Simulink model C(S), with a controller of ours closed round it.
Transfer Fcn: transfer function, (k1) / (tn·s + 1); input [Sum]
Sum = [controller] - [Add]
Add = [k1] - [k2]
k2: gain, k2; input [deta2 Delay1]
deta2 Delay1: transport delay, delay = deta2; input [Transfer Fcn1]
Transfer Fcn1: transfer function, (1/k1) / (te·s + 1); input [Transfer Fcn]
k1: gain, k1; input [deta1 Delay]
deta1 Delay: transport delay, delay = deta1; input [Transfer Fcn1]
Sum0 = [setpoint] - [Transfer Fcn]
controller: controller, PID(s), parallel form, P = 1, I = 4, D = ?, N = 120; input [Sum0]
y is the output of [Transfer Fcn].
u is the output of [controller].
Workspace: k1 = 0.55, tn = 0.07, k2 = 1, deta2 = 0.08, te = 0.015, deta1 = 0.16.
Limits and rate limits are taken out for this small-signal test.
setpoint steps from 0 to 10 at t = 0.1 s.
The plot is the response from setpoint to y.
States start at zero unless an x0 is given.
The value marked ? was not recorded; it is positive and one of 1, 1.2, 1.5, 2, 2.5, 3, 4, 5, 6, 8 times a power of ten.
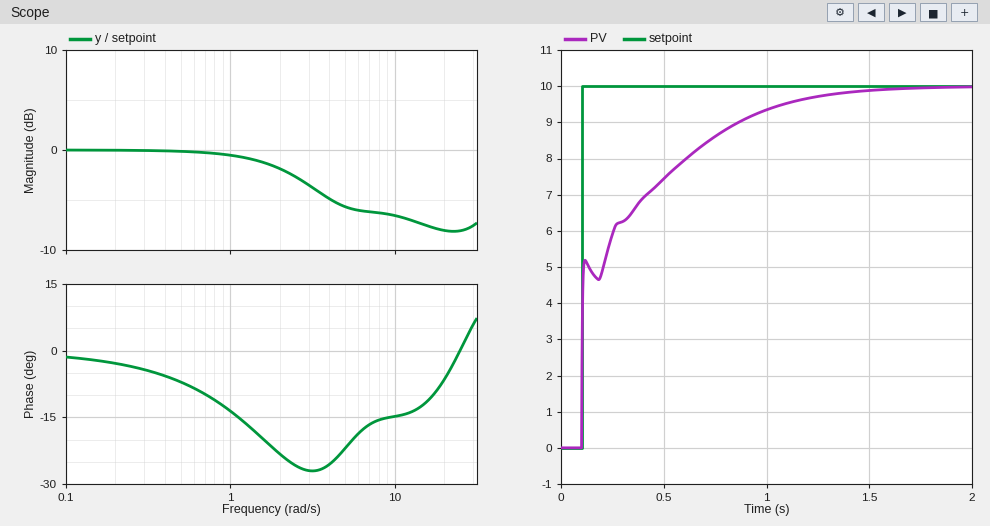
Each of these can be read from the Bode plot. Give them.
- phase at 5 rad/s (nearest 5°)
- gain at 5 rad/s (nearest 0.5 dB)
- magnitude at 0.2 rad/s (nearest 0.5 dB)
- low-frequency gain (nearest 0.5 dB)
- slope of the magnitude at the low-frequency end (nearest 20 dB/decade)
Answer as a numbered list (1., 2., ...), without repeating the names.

1. -20°
2. -5.5 dB
3. 0.0 dB
4. 0.0 dB
5. 0 dB/decade
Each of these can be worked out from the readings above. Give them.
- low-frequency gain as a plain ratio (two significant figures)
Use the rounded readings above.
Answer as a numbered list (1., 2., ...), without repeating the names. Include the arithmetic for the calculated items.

1. 10^(0 / 20) = 1.0
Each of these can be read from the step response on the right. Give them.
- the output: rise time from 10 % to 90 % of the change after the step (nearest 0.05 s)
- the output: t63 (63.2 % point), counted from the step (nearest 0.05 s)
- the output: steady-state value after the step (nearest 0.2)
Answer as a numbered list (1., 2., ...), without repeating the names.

1. 0.75 s
2. 0.20 s
3. 10.0
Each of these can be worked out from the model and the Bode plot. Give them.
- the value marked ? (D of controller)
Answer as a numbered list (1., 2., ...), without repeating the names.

1. 0.15
